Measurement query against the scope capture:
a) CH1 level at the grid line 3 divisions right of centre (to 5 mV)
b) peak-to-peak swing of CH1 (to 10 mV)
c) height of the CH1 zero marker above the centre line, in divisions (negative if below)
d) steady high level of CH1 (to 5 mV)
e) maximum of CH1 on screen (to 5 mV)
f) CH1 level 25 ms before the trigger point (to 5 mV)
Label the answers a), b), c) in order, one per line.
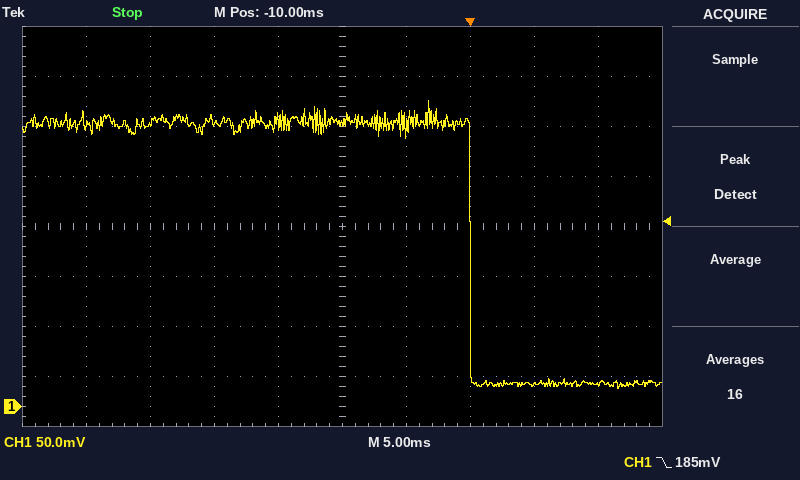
a) 20 mV
b) 290 mV
c) -3.6 div
d) 285 mV
e) 305 mV
f) 285 mV
